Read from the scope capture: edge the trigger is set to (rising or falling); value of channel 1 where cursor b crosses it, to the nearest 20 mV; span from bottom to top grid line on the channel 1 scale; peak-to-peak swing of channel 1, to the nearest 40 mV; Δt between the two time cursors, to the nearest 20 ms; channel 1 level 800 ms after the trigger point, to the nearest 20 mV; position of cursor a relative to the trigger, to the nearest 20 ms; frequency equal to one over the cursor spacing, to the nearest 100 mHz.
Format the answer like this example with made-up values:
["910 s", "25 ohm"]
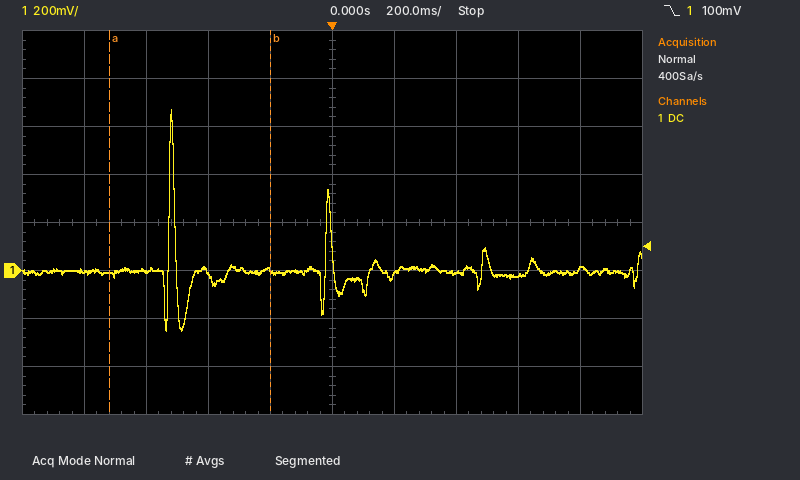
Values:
["falling", "0 mV", "1.6 V", "920 mV", "520 ms", "0 mV", "-720 ms", "1.9 Hz"]
